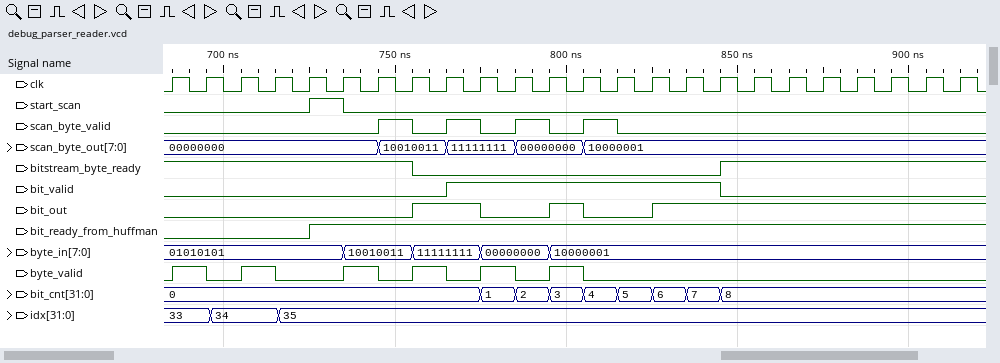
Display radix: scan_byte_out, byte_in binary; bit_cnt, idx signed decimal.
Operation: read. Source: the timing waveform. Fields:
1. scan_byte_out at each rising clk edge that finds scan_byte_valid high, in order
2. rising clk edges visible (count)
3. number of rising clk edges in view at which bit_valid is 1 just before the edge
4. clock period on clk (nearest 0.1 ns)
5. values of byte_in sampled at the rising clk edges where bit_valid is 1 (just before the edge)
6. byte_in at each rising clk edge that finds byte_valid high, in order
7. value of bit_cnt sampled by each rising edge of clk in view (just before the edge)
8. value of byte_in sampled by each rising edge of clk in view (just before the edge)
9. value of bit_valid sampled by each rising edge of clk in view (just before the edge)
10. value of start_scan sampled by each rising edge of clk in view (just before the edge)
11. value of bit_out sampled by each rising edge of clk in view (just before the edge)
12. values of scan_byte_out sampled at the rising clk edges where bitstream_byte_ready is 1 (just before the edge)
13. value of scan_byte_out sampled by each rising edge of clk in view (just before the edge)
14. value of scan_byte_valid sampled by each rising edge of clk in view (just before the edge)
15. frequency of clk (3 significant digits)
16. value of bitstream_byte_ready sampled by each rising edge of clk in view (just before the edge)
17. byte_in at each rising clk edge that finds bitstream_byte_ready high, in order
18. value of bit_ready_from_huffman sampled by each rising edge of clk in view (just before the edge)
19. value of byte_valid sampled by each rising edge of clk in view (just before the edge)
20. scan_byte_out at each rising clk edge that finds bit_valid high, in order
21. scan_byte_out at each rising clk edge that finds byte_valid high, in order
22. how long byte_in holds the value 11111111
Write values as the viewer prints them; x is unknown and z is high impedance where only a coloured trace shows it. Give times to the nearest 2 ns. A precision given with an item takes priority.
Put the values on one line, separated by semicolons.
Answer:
10010011, 11111111, 00000000, 10000001; 24; 8; 10 ns; 11111111, 00000000, 00000000, 10000001, 10000001, 10000001, 10000001, 10000001; 01010101, 01010101, 10010011, 11111111, 00000000, 10000001; 0, 0, 0, 0, 0, 0, 0, 0, 0, 0, 1, 2, 3, 4, 5, 6, 7, 8, 8, 8, 8, 8, 8, 8; 01010101, 01010101, 01010101, 01010101, 01010101, 01010101, 10010011, 10010011, 11111111, 11111111, 00000000, 00000000, 10000001, 10000001, 10000001, 10000001, 10000001, 10000001, 10000001, 10000001, 10000001, 10000001, 10000001, 10000001; 0 0 0 0 0 0 0 0 0 1 1 1 1 1 1 1 1 0 0 0 0 0 0 0; 0 0 0 0 0 1 0 0 0 0 0 0 0 0 0 0 0 0 0 0 0 0 0 0; 0 0 0 0 0 0 0 0 1 1 0 0 1 0 0 1 1 1 1 1 1 1 1 1; 00000000, 00000000, 00000000, 00000000, 00000000, 00000000, 00000000, 10010011, 10000001, 10000001, 10000001, 10000001, 10000001, 10000001, 10000001; 00000000, 00000000, 00000000, 00000000, 00000000, 00000000, 00000000, 10010011, 10010011, 11111111, 11111111, 00000000, 00000000, 10000001, 10000001, 10000001, 10000001, 10000001, 10000001, 10000001, 10000001, 10000001, 10000001, 10000001; 0 0 0 0 0 0 0 1 0 1 0 1 0 1 0 0 0 0 0 0 0 0 0 0; 100 MHz; 1 1 1 1 1 1 1 1 0 0 0 0 0 0 0 0 0 1 1 1 1 1 1 1; 01010101, 01010101, 01010101, 01010101, 01010101, 01010101, 10010011, 10010011, 10000001, 10000001, 10000001, 10000001, 10000001, 10000001, 10000001; 0 0 0 0 0 1 1 1 1 1 1 1 1 1 1 1 1 1 1 1 1 1 1 1; 0 1 0 1 0 0 1 0 1 0 1 0 1 0 0 0 0 0 0 0 0 0 0 0; 11111111, 11111111, 00000000, 00000000, 10000001, 10000001, 10000001, 10000001; 00000000, 00000000, 00000000, 10010011, 11111111, 00000000; 20 ns
